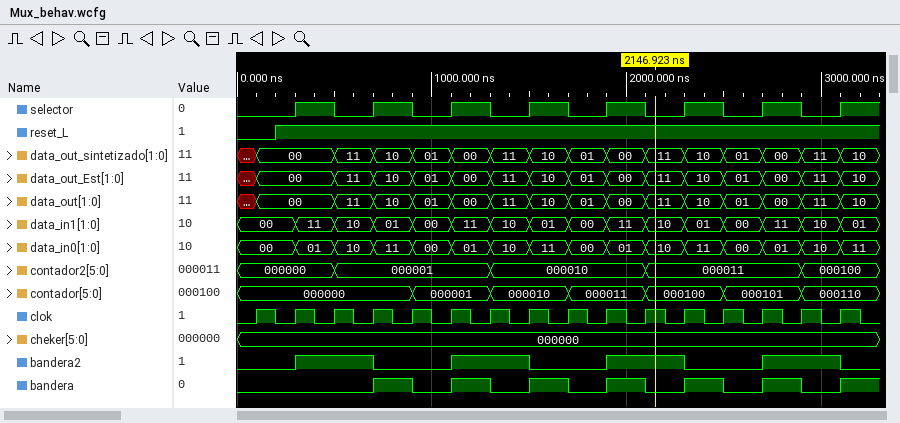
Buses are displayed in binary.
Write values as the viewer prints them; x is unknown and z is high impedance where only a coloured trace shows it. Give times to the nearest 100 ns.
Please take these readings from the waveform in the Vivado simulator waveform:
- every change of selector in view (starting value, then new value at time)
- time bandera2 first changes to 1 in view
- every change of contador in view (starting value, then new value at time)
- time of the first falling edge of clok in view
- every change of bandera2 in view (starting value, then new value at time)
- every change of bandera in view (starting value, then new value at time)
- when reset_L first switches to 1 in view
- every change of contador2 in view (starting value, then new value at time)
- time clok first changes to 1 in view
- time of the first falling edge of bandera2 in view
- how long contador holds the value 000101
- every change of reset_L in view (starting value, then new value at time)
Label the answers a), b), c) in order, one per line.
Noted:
a) 0, 1 at 300 ns, 0 at 500 ns, 1 at 700 ns, 0 at 900 ns, 1 at 1100 ns, 0 at 1300 ns, 1 at 1500 ns, 0 at 1700 ns, 1 at 1900 ns, 0 at 2100 ns, 1 at 2300 ns, 0 at 2500 ns, 1 at 2700 ns, 0 at 2900 ns, 1 at 3100 ns
b) 300 ns
c) 000000, 000001 at 900 ns, 000010 at 1300 ns, 000011 at 1700 ns, 000100 at 2100 ns, 000101 at 2500 ns, 000110 at 2900 ns
d) 200 ns
e) 0, 1 at 300 ns, 0 at 700 ns, 1 at 1100 ns, 0 at 1500 ns, 1 at 1900 ns, 0 at 2300 ns, 1 at 2700 ns, 0 at 3100 ns
f) 0, 1 at 700 ns, 0 at 900 ns, 1 at 1100 ns, 0 at 1300 ns, 1 at 1500 ns, 0 at 1700 ns, 1 at 1900 ns, 0 at 2100 ns, 1 at 2300 ns, 0 at 2500 ns, 1 at 2700 ns, 0 at 2900 ns, 1 at 3100 ns
g) 200 ns
h) 000000, 000001 at 500 ns, 000010 at 1300 ns, 000011 at 2100 ns, 000100 at 2900 ns
i) 100 ns
j) 700 ns
k) 400 ns
l) 0, 1 at 200 ns
